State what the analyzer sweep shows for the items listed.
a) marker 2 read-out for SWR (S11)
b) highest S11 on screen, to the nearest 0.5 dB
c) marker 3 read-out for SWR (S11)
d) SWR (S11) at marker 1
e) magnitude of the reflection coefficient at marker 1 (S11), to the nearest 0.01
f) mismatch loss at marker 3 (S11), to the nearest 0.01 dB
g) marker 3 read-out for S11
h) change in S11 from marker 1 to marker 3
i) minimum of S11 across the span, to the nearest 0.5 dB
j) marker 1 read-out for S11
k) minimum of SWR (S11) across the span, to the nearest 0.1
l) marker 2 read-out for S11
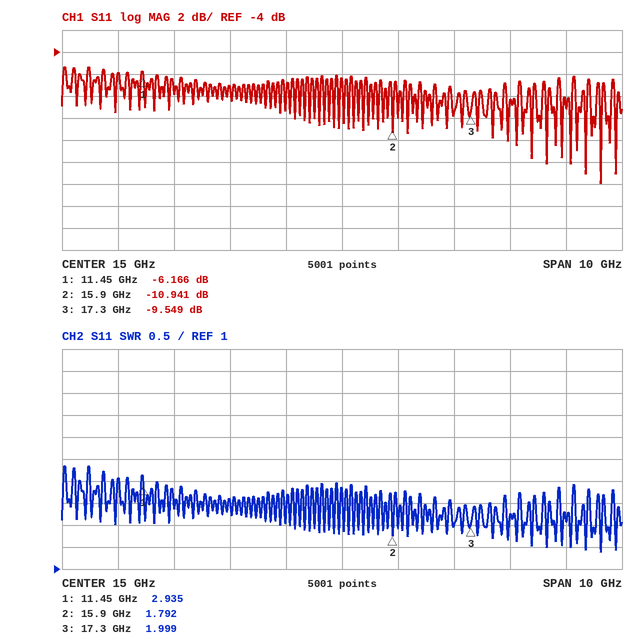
1.792
-5.5 dB
1.999
2.935
0.49
0.51 dB
-9.549 dB
-3.383 dB
-16.0 dB
-6.166 dB
1.4
-10.941 dB
